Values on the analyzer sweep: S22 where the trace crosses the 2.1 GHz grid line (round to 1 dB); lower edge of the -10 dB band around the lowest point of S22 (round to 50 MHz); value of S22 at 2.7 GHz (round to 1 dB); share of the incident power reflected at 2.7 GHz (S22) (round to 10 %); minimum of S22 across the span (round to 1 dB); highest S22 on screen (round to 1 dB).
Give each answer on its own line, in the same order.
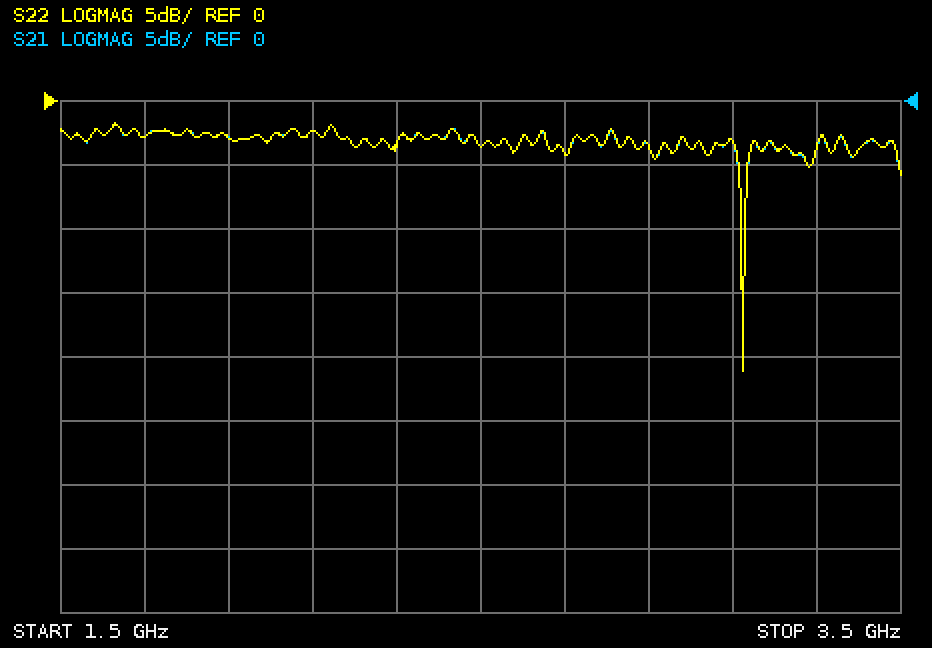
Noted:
-2 dB
3.10 GHz
-4 dB
40 %
-21 dB
-2 dB
